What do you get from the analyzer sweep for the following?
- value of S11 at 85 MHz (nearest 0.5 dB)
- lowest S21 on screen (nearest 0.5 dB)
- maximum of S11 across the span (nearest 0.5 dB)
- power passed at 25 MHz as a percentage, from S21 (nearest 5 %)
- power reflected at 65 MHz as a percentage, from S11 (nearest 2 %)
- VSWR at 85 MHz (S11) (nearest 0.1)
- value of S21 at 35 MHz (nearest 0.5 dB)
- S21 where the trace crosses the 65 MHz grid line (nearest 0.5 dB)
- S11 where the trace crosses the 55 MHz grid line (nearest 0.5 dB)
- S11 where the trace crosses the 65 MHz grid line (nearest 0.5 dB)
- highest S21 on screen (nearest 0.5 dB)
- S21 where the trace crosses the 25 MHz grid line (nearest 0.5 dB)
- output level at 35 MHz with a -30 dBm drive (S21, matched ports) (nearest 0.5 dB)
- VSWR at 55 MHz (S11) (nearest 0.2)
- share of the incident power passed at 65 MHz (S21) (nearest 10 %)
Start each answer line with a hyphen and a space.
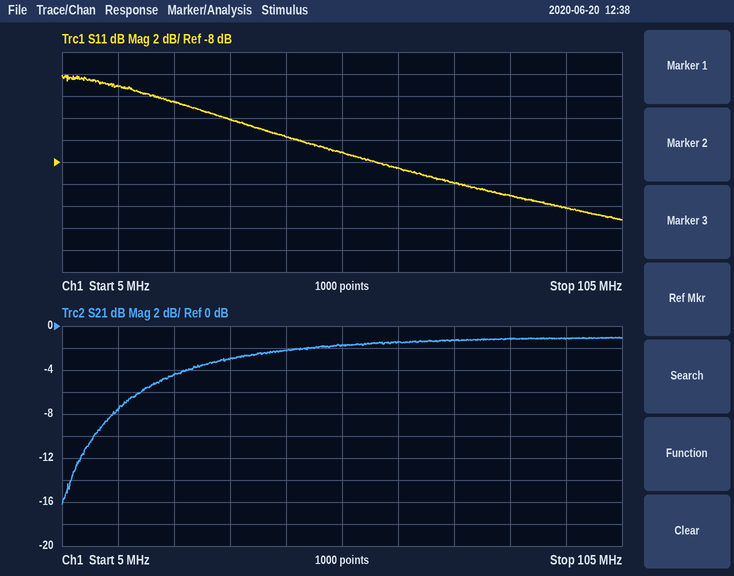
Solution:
- -11.0 dB
- -16.0 dB
- 0.0 dB
- 35 %
- 14 %
- 1.8
- -3.0 dB
- -1.5 dB
- -7.0 dB
- -8.5 dB
- -1.0 dB
- -4.5 dB
- -33.0 dBm
- 2.6
- 70 %
